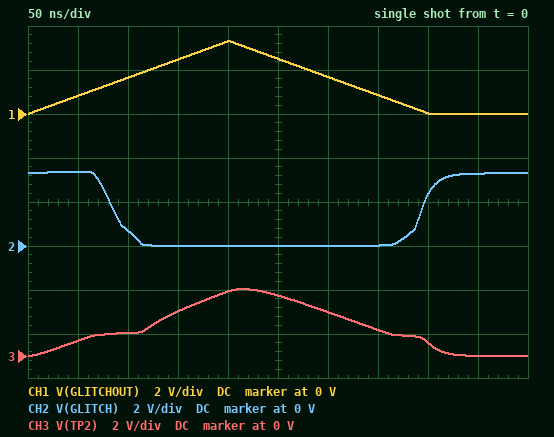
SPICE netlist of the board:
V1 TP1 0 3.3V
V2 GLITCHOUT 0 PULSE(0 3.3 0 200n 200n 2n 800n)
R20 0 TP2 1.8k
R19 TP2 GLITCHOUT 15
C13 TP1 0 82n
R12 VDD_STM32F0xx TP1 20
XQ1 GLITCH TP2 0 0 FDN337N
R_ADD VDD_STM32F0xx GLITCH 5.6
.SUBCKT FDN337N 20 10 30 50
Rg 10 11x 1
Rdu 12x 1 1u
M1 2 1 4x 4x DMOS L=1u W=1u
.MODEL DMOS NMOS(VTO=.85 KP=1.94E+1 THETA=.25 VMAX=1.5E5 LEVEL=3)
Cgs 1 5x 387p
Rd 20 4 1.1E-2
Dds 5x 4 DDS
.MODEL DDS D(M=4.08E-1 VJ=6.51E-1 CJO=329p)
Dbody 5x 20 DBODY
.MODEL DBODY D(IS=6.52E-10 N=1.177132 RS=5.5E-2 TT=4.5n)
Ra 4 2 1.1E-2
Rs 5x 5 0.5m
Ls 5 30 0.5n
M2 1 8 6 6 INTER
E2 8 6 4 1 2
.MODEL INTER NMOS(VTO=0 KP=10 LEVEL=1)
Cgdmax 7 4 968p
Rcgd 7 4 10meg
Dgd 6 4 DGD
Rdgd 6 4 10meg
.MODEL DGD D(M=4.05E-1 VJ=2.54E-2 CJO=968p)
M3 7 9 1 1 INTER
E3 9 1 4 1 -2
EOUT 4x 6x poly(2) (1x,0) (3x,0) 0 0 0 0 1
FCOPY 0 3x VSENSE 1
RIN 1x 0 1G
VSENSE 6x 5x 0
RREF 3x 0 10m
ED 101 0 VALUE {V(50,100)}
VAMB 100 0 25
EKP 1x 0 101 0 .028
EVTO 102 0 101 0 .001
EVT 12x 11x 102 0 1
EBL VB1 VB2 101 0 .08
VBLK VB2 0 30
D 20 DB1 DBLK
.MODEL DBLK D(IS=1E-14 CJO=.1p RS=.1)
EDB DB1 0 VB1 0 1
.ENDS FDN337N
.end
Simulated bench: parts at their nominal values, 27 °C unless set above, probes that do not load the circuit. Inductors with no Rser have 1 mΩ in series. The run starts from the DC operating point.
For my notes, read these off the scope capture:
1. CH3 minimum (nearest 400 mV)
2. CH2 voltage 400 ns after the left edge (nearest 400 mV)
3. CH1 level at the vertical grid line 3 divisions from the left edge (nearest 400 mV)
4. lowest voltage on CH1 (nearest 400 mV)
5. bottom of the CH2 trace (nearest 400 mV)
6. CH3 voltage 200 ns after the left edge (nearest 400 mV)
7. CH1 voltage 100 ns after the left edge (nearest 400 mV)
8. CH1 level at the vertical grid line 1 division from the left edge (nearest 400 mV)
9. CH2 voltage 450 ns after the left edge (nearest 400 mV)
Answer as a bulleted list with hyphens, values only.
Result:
- 0 V
- 2.4 V
- 2.4 V
- 0 V
- 0 V
- 2.8 V
- 1.6 V
- 800 mV
- 3.2 V
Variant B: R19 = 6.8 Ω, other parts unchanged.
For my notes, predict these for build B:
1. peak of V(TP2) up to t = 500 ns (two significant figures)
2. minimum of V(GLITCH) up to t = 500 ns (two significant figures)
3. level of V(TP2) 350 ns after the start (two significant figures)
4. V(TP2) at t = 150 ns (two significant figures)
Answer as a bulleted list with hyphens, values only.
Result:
- 3.2 V
- 5.3 mV
- 1.0 V
- 2.3 V
